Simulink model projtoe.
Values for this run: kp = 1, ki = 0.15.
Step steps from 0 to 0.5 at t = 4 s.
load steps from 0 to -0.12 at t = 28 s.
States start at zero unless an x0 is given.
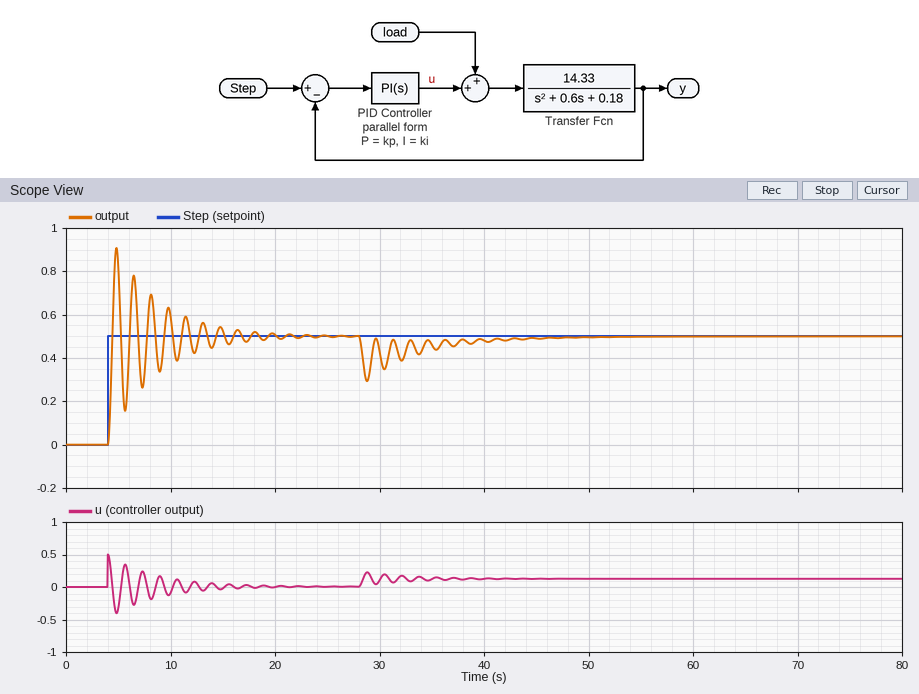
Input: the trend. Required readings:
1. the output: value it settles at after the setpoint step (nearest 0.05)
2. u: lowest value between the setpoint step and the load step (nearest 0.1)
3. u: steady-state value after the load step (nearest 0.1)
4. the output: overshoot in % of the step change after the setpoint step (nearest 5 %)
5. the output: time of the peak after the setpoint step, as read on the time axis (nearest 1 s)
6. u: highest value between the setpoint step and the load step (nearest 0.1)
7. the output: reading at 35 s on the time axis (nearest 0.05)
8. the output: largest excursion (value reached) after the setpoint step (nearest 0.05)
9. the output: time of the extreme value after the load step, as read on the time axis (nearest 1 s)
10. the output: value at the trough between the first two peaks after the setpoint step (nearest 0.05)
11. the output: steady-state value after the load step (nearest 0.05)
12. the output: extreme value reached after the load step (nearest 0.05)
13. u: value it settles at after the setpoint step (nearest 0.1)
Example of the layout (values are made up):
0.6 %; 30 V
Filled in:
0.50; -0.4; 0.1; 80 %; 5 s; 0.5; 0.45; 0.90; 29 s; 0.15; 0.50; 0.30; 0.0
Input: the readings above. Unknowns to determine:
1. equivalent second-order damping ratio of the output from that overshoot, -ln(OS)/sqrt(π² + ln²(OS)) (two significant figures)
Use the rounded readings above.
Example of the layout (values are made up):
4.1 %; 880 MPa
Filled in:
0.071
